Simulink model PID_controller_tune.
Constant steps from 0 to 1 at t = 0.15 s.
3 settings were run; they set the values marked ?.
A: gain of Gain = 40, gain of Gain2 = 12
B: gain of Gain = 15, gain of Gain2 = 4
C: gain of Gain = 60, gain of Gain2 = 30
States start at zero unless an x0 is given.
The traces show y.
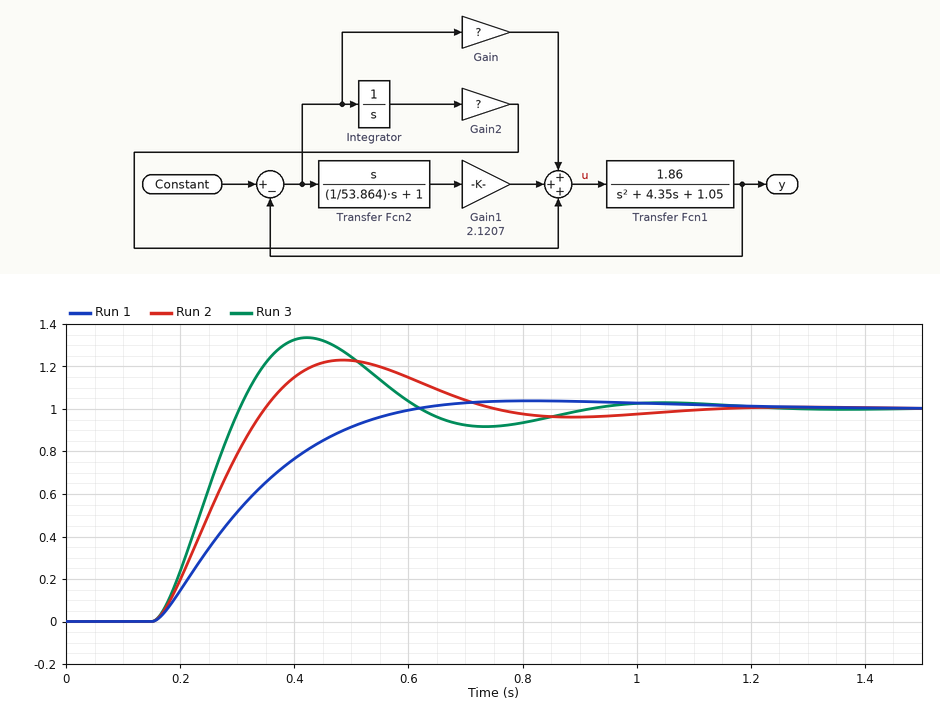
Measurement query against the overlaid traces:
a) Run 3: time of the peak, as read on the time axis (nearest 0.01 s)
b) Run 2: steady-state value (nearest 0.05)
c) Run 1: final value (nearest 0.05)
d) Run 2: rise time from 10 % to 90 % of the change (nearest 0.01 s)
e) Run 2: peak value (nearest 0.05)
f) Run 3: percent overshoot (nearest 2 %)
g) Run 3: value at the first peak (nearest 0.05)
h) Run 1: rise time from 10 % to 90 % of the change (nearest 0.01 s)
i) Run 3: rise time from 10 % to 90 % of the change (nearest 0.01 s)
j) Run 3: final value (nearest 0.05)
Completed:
0.42 s
1.00
1.00
0.14 s
1.25
34 %
1.35
0.30 s
0.11 s
1.00
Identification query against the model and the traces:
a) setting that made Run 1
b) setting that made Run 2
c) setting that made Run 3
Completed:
B
A
C
